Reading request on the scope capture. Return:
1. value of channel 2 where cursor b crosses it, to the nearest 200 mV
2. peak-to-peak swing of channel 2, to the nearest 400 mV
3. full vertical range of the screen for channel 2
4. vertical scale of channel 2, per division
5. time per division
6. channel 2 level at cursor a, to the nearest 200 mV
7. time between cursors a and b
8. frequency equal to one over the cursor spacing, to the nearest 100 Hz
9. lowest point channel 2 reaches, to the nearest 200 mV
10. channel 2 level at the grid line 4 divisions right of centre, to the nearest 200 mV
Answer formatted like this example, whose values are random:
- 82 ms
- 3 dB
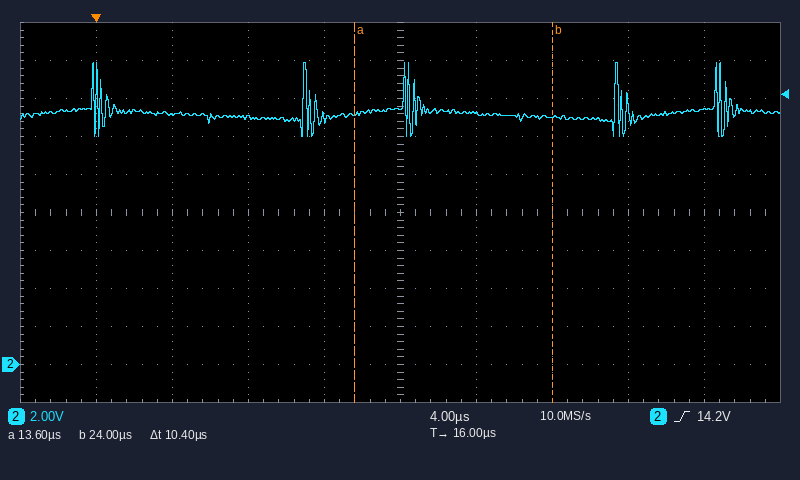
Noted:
- 13.0 V
- 4.0 V
- 20 V
- 2 V
- 4 µs
- 13.2 V
- 10.4 µs
- 96.2 kHz
- 12.0 V
- 13.4 V
